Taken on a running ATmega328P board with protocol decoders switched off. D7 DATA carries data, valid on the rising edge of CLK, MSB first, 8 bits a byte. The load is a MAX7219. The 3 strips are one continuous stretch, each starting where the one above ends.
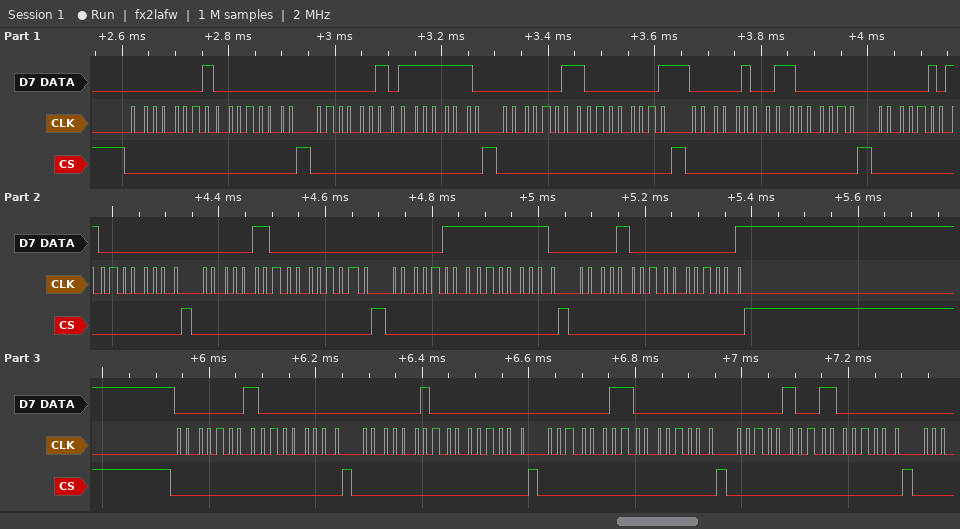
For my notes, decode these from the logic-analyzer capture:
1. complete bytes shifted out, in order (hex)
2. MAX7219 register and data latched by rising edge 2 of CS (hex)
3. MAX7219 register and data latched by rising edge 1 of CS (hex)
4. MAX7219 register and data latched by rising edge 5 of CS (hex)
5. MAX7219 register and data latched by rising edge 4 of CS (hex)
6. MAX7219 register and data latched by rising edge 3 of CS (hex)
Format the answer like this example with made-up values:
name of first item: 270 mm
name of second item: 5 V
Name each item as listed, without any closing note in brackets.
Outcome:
complete bytes shifted out, in order: 01 00 02 FE 03 01 04 C0 05 00 06 00 07 FE 08 01 01 00 02 00 03 00 04 C0
MAX7219 register and data latched by rising edge 2 of CS: register 0x2, data 0xFE
MAX7219 register and data latched by rising edge 1 of CS: register 0x1, data 0x00
MAX7219 register and data latched by rising edge 5 of CS: register 0x5, data 0x00
MAX7219 register and data latched by rising edge 4 of CS: register 0x4, data 0xC0
MAX7219 register and data latched by rising edge 3 of CS: register 0x3, data 0x01
